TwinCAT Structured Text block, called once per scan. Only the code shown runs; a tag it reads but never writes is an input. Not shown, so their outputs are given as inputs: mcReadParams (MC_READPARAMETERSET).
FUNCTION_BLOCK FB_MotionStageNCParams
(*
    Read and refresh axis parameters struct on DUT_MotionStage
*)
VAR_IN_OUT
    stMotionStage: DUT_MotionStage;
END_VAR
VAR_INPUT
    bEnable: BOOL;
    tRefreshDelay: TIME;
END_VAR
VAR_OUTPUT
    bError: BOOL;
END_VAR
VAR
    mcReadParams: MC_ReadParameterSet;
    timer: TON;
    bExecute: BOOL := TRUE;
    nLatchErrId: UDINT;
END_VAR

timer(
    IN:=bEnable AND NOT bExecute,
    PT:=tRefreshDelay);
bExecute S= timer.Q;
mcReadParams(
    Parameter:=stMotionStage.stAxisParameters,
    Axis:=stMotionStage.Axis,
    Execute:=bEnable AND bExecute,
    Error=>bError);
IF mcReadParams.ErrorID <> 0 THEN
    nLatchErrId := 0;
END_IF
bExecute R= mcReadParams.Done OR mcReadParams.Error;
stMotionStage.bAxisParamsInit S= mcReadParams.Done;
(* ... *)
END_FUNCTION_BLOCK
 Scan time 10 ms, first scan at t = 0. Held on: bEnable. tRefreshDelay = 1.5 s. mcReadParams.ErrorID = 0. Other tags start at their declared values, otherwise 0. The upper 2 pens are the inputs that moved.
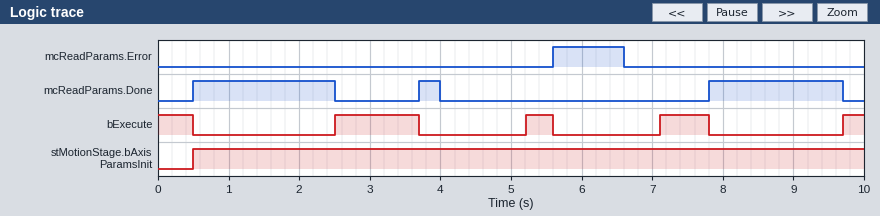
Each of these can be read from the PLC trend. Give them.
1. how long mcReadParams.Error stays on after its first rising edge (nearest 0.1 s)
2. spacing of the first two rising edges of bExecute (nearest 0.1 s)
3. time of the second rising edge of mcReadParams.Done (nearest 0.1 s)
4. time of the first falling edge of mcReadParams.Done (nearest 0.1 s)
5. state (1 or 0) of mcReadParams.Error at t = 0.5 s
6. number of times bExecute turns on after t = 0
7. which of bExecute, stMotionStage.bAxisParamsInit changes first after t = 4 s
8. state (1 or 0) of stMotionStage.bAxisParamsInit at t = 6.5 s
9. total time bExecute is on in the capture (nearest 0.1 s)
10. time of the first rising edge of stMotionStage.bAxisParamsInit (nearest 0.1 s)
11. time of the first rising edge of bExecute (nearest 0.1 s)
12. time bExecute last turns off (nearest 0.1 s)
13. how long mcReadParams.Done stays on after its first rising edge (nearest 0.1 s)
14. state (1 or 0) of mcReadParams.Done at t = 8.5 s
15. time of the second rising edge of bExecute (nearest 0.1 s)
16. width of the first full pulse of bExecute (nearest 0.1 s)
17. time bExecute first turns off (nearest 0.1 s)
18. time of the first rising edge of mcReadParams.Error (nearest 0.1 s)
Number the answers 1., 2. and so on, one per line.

1. 1.0 s
2. 2.7 s
3. 3.7 s
4. 2.5 s
5. 0
6. 4
7. bExecute
8. 1
9. 3.1 s
10. 0.5 s
11. 2.5 s
12. 7.8 s
13. 2.0 s
14. 1
15. 5.2 s
16. 1.2 s
17. 0.5 s
18. 5.6 s
